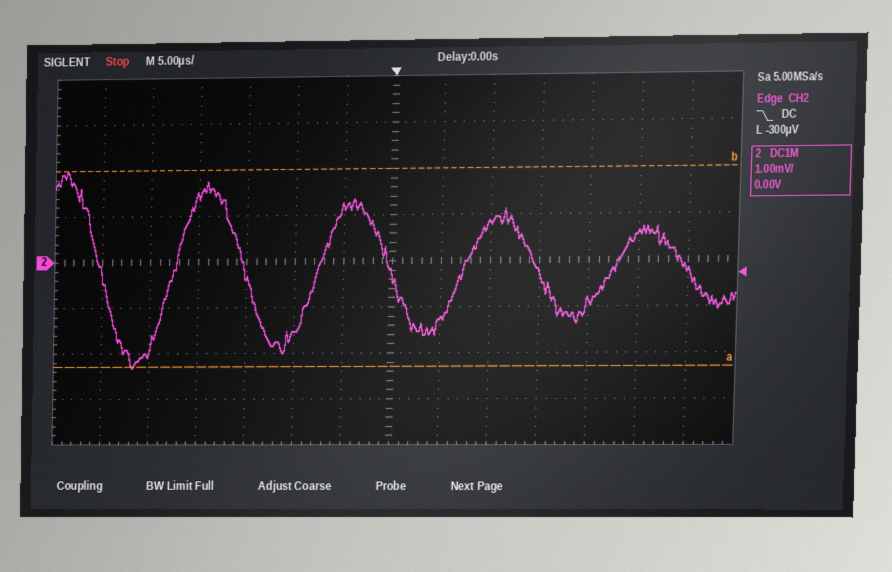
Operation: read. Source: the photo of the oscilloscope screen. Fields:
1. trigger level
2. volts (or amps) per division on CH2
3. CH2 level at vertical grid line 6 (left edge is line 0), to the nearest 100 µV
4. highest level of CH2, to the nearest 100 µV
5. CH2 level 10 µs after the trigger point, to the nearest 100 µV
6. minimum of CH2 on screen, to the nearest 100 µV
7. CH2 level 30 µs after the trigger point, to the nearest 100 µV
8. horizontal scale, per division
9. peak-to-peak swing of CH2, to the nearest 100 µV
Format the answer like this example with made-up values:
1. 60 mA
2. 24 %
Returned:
1. -300 µV
2. 1 mV
3. 1.2 mV
4. 2.0 mV
5. 800 µV
6. -2.3 mV
7. -200 µV
8. 5 µs
9. 4.3 mV
